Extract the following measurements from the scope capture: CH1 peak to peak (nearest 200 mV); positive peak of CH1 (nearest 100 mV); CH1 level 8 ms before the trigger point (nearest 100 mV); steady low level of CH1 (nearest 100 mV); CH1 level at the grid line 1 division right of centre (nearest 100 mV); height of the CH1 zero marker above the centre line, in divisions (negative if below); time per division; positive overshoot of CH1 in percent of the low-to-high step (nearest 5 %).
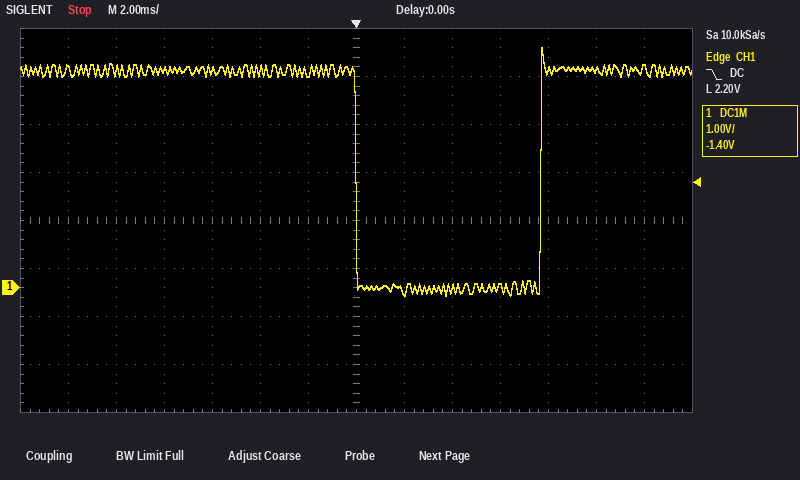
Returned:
5.2 V
5.0 V
4.5 V
0.0 V
-100 mV
-1.4 div
2 ms
10 %
